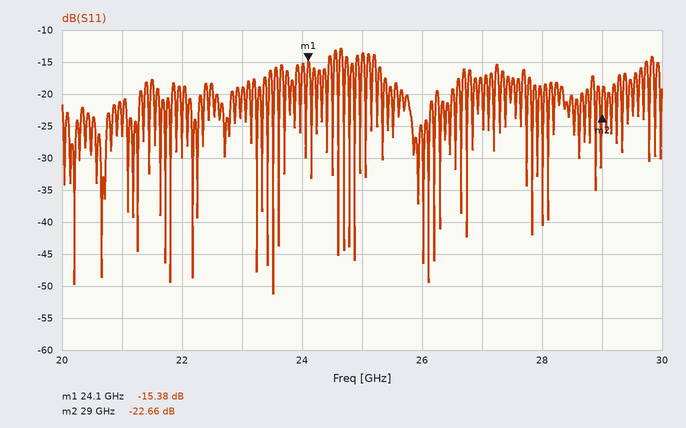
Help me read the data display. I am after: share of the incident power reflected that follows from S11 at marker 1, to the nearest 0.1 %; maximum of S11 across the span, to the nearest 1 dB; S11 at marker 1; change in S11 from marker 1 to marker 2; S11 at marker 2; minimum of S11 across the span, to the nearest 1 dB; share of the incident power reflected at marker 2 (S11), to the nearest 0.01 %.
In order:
2.9 %
-13 dB
-15.38 dB
-7.28 dB
-22.66 dB
-51 dB
0.54 %
